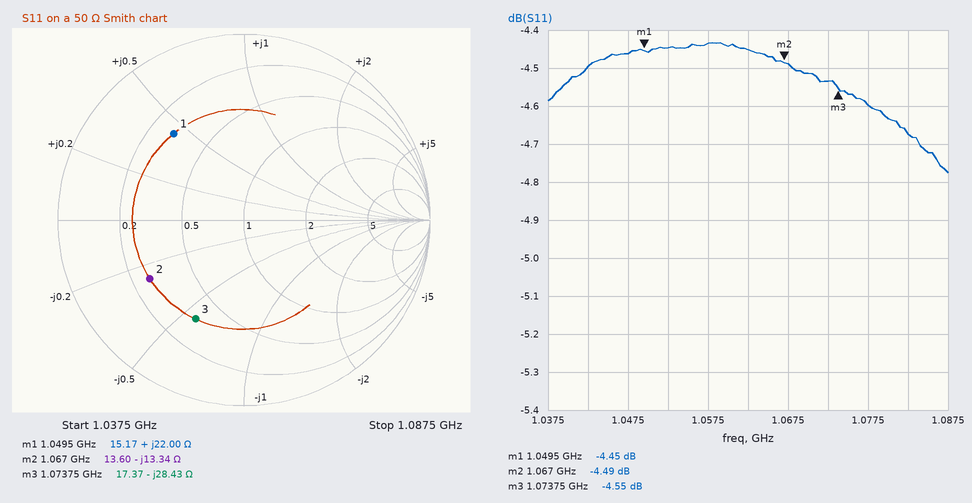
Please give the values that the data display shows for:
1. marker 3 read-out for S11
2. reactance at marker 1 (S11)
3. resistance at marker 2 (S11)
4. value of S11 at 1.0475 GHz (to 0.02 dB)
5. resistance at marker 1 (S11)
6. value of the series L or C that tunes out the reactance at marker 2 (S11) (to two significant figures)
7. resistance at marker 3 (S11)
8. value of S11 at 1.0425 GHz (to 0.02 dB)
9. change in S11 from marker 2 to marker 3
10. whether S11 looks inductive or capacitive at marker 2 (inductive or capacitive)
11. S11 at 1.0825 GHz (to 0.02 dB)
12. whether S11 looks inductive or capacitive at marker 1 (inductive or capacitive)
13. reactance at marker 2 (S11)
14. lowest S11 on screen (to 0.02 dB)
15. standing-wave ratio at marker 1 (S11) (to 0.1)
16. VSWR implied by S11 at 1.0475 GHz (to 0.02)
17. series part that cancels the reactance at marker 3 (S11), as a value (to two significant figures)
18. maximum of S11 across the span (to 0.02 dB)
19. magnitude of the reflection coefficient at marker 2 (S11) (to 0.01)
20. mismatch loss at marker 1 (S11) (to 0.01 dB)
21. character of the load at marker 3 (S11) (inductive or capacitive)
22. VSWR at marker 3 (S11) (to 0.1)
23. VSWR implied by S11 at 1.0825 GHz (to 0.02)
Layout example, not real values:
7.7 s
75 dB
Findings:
-4.55 dB
+22.00 Ω
13.60 Ω
-4.46 dB
15.17 Ω
2.0 nH
17.37 Ω
-4.50 dB
-0.06 dB
capacitive
-4.68 dB
inductive
-13.34 Ω
-4.78 dB
4.0
3.98
4.2 nH
-4.44 dB
0.60
1.93 dB
capacitive
3.9
3.80
